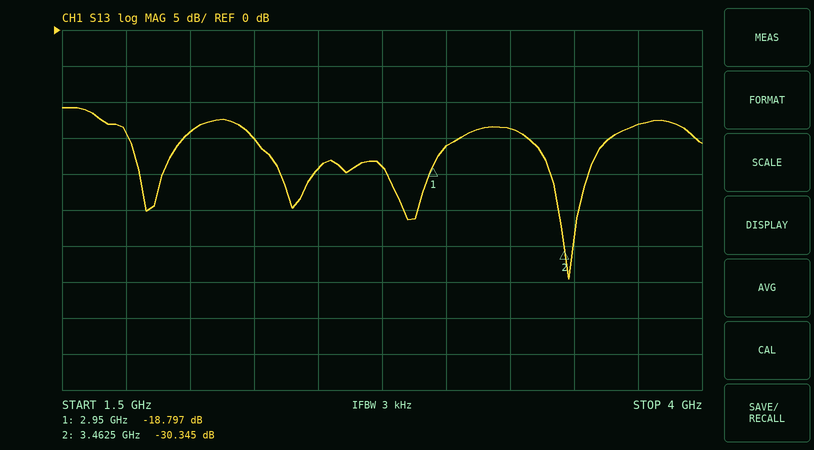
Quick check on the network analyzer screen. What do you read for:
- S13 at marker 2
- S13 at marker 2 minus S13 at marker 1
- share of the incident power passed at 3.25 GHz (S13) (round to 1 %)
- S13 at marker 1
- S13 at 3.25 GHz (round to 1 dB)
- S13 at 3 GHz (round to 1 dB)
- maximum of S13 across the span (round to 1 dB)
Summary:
-30.345 dB
-11.548 dB
4 %
-18.797 dB
-14 dB
-16 dB
-11 dB
